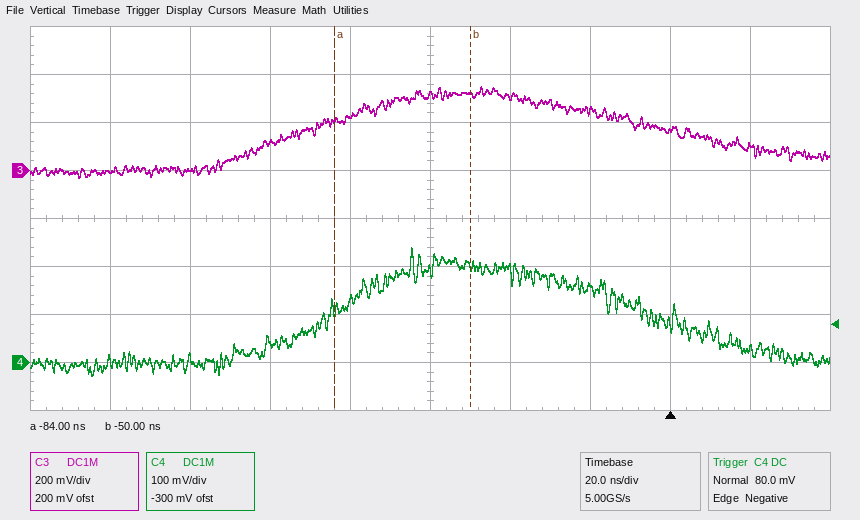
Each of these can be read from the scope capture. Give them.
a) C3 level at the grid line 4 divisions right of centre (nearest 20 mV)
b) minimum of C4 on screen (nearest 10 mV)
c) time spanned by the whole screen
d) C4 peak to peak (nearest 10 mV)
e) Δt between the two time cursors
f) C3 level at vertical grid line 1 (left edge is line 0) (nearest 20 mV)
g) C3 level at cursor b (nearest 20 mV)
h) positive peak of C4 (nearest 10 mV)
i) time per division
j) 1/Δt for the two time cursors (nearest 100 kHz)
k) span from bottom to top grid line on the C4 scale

100 mV
-30 mV
200 ns
270 mV
34 ns
0 mV
320 mV
240 mV
20 ns
29.4 MHz
800 mV
